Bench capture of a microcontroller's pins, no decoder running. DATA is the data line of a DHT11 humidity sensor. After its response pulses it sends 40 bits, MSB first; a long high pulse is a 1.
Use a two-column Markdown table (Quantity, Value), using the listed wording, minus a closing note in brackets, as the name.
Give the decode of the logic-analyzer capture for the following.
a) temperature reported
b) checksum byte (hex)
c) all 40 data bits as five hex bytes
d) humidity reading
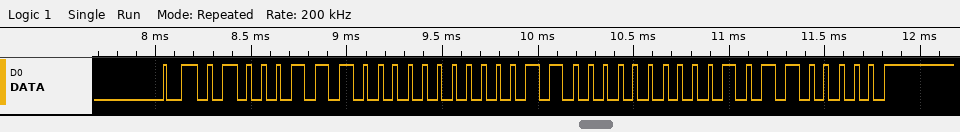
| Quantity | Value |
|---|---|
| temperature reported | 24.1 °C |
| checksum byte | 0x60 |
| all 40 data bits as five hex bytes | 47 00 18 01 60 |
| humidity reading | 71 % |
